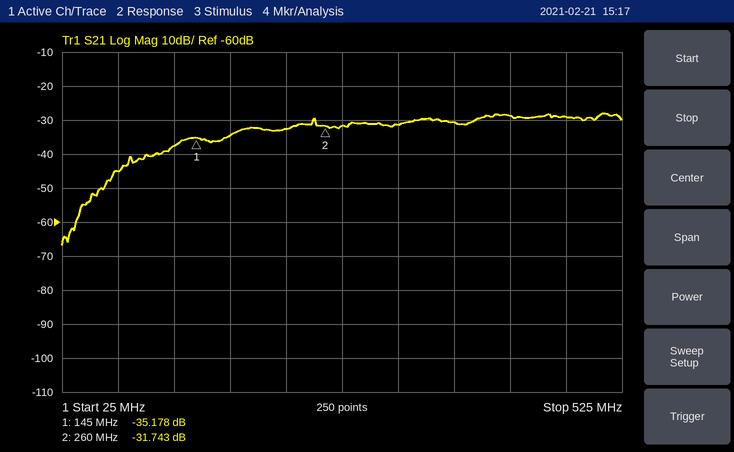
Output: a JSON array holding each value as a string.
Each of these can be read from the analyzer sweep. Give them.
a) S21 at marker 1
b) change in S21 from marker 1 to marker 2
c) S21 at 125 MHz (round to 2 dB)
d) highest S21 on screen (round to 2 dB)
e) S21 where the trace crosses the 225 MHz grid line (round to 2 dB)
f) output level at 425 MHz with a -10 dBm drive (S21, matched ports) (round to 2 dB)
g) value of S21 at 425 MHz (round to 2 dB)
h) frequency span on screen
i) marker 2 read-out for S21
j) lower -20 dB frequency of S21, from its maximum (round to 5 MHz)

["-35.178 dB", "3.435 dB", "-38 dB", "-28 dB", "-32 dB", "-38 dBm", "-28 dB", "500 MHz", "-31.743 dB", "65 MHz"]
